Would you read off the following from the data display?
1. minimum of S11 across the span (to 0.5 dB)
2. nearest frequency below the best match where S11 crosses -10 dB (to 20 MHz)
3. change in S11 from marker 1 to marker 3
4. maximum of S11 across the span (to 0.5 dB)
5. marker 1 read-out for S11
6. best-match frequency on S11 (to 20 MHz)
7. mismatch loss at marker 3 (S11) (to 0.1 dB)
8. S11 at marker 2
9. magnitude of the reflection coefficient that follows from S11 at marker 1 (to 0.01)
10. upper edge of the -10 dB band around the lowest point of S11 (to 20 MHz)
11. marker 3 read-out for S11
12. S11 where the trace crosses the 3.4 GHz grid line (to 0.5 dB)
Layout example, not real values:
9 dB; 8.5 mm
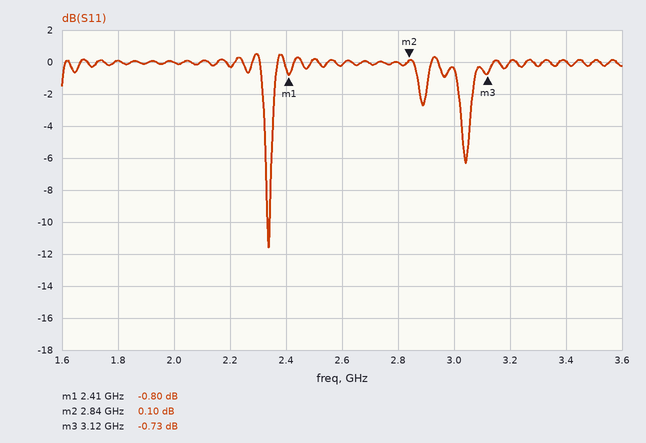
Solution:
-11.5 dB; 2.34 GHz; 0.07 dB; 0.5 dB; -0.80 dB; 2.34 GHz; 8.1 dB; 0.10 dB; 0.91; 2.34 GHz; -0.73 dB; 0.0 dB
